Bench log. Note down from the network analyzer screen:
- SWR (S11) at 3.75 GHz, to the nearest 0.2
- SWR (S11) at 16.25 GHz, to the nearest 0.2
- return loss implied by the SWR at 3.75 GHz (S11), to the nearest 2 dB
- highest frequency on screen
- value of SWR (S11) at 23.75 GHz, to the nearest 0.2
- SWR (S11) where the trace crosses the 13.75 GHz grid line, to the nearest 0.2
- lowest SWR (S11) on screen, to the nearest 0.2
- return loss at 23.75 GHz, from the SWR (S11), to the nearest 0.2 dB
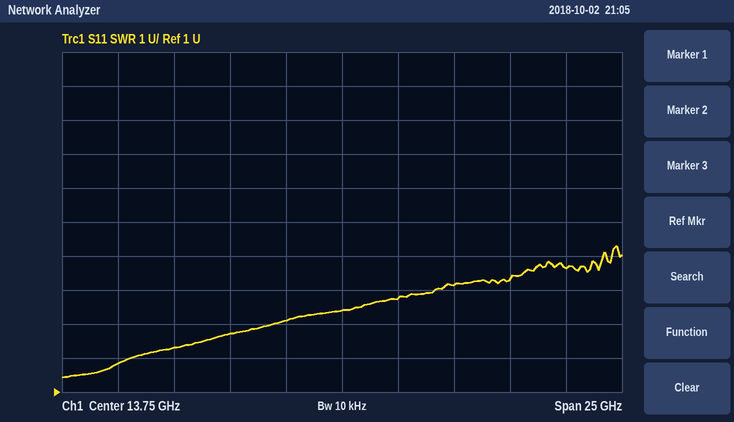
1.8
3.8
10 dB
26.25 GHz
4.6
3.4
1.4
3.8 dB
